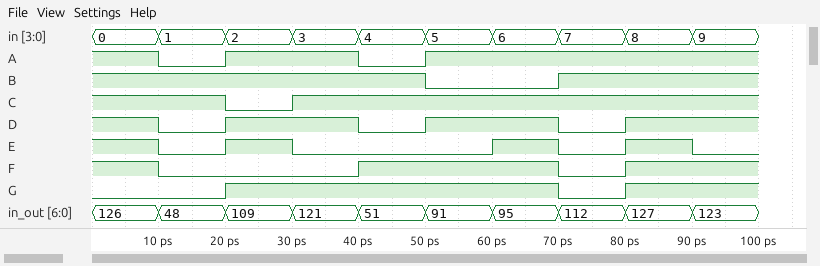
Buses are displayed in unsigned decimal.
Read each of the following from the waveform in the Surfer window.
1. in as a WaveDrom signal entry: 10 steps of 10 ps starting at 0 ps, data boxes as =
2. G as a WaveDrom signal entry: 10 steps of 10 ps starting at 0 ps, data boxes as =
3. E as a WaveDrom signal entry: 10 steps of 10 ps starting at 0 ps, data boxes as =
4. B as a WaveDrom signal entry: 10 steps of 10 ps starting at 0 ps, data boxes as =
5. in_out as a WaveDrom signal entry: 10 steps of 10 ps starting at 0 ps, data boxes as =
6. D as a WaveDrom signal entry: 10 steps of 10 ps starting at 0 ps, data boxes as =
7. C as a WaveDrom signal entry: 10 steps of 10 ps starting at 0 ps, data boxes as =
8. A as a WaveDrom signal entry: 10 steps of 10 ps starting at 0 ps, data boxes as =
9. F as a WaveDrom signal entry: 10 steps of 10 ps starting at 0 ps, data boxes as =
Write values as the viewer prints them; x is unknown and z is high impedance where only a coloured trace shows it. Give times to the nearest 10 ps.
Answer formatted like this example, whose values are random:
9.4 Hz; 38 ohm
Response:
{name: 'in', wave: '==========', data: '0 1 2 3 4 5 6 7 8 9'}; {name: 'G', wave: '0.1....01.'}; {name: 'E', wave: '1010..1010'}; {name: 'B', wave: '1....0.1..'}; {name: 'in_out', wave: '==========', data: '126 48 109 121 51 91 95 112 127 123'}; {name: 'D', wave: '101.01.01.'}; {name: 'C', wave: '1.01......'}; {name: 'A', wave: '101.01....'}; {name: 'F', wave: '10..1..01.'}
